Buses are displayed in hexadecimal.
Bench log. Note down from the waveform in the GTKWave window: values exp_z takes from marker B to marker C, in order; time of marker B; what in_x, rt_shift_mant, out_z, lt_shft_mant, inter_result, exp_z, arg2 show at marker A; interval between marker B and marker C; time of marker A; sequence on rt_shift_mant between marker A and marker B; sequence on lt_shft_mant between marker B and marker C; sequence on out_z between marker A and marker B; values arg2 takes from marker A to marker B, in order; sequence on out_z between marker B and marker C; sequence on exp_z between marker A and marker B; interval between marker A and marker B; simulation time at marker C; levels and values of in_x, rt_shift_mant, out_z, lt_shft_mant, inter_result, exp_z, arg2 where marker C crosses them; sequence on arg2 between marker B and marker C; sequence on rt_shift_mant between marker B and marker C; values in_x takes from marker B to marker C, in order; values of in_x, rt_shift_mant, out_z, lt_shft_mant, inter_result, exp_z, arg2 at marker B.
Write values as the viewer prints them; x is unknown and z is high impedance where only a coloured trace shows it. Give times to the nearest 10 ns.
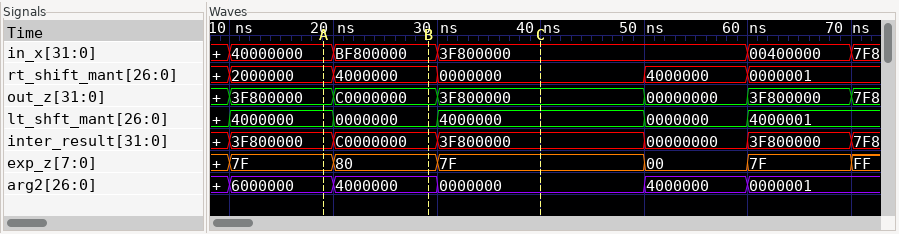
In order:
80, 7F
30 ns
in_x=40000000, rt_shift_mant=2000000, out_z=3F800000, lt_shft_mant=4000000, inter_result=3F800000, exp_z=7F, arg2=6000000
10 ns
20 ns
2000000, 4000000
0000000, 4000000
3F800000, C0000000
6000000, 4000000
C0000000, 3F800000
7F, 80
10 ns
40 ns
in_x=3F800000, rt_shift_mant=0000000, out_z=3F800000, lt_shft_mant=4000000, inter_result=3F800000, exp_z=7F, arg2=0000000
4000000, 0000000
4000000, 0000000
BF800000, 3F800000
in_x=BF800000, rt_shift_mant=4000000, out_z=C0000000, lt_shft_mant=0000000, inter_result=C0000000, exp_z=80, arg2=4000000
